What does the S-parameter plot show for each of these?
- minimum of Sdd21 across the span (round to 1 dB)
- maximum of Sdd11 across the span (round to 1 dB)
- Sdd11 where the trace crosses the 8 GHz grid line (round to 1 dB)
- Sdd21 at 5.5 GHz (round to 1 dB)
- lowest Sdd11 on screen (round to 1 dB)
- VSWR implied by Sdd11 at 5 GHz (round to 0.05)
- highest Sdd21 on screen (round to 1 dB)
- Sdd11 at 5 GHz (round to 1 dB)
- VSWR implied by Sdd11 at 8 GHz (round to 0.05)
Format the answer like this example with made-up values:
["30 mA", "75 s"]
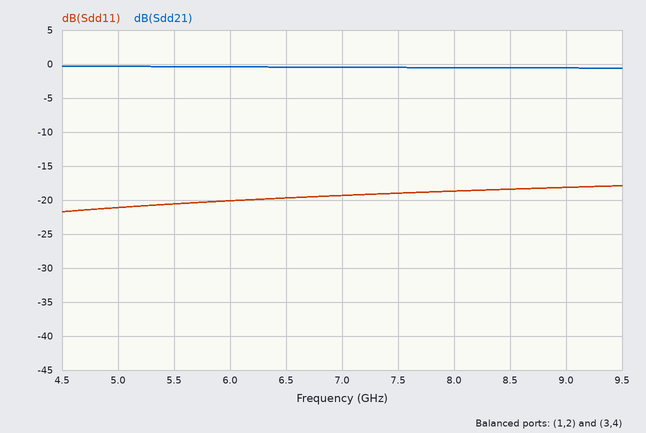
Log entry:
["-1 dB", "-18 dB", "-19 dB", "0 dB", "-22 dB", "1.20", "0 dB", "-21 dB", "1.25"]
